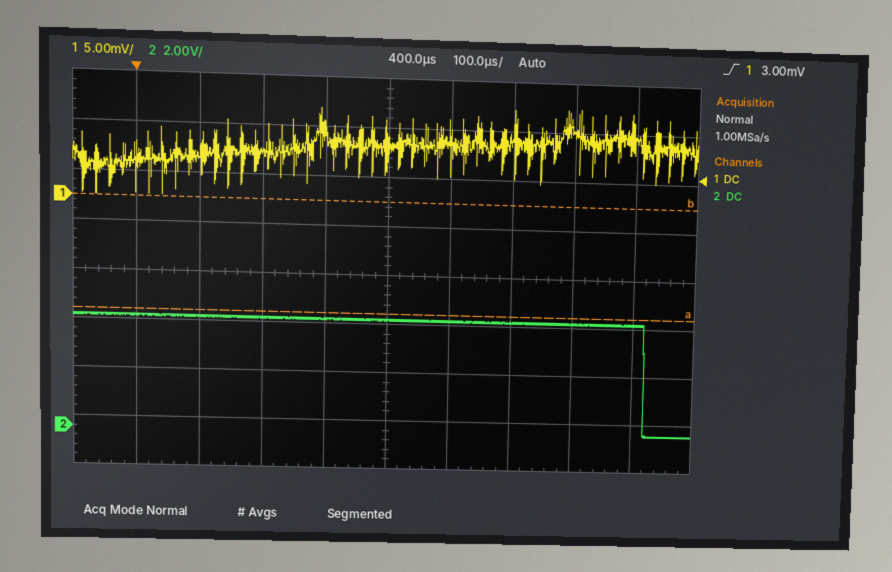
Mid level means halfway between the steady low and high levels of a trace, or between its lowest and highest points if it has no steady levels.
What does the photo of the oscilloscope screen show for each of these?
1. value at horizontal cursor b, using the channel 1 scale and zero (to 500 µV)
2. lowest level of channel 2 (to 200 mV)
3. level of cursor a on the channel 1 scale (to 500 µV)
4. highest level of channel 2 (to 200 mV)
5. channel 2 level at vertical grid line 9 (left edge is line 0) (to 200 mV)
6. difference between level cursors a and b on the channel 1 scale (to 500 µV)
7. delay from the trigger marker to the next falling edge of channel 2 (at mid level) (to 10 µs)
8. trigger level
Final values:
0.0 mV
0.0 V
-11.5 mV
4.6 V
4.6 V
11.5 mV
820 µs
3.00 mV
